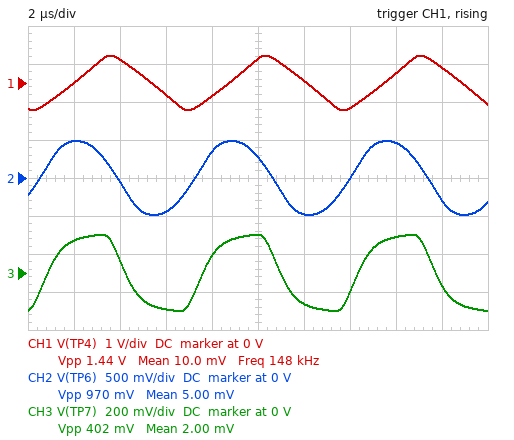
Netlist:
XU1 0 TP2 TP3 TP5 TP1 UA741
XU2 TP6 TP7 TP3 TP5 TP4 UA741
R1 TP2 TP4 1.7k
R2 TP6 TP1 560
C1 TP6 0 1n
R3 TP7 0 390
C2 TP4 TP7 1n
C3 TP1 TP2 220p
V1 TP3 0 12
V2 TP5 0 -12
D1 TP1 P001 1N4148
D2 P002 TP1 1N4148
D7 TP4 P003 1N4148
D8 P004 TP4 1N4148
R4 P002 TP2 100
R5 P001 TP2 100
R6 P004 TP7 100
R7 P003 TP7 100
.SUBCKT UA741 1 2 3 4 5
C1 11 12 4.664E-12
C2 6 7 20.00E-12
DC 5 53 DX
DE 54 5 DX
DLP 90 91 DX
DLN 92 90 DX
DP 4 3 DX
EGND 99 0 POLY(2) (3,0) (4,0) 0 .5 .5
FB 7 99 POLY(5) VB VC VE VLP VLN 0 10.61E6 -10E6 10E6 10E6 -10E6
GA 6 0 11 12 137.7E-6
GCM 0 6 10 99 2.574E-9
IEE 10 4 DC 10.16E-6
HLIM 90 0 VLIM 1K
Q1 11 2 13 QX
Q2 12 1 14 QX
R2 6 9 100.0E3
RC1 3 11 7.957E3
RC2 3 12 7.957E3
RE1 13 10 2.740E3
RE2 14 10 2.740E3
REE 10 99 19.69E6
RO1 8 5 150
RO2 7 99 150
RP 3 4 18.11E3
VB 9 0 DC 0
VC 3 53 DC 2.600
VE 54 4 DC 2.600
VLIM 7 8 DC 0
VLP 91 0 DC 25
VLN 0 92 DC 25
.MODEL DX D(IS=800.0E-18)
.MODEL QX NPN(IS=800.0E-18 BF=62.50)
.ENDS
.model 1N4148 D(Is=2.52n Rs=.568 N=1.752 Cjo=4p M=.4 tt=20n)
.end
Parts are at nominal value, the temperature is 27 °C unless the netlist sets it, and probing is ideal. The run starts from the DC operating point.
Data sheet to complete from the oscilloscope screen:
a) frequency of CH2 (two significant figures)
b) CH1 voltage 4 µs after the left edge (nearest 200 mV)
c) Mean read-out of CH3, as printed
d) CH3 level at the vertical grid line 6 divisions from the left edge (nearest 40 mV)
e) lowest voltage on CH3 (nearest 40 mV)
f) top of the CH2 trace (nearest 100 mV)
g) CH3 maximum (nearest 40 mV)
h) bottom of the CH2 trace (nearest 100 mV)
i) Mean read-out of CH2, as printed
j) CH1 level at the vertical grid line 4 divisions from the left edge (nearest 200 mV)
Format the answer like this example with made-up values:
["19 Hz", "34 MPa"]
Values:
["150 kHz", "600 mV", "2.00 mV", "-160 mV", "-200 mV", "500 mV", "200 mV", "-500 mV", "5.00 mV", "-400 mV"]
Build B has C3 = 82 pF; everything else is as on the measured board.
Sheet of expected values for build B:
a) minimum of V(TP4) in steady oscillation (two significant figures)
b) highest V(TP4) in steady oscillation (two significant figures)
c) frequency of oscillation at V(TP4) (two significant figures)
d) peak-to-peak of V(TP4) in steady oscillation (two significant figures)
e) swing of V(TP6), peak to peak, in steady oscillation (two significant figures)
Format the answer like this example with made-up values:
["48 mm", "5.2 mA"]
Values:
["-660 mV", "660 mV", "160 kHz", "1.3 V", "950 mV"]
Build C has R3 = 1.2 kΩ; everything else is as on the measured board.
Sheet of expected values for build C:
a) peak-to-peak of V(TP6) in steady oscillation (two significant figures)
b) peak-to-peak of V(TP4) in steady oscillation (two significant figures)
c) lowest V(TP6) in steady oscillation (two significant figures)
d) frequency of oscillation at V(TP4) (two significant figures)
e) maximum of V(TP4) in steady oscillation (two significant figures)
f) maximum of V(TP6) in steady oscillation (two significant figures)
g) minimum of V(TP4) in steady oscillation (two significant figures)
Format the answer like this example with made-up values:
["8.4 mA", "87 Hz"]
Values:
["780 mV", "790 mV", "-390 mV", "190 kHz", "400 mV", "390 mV", "-400 mV"]
